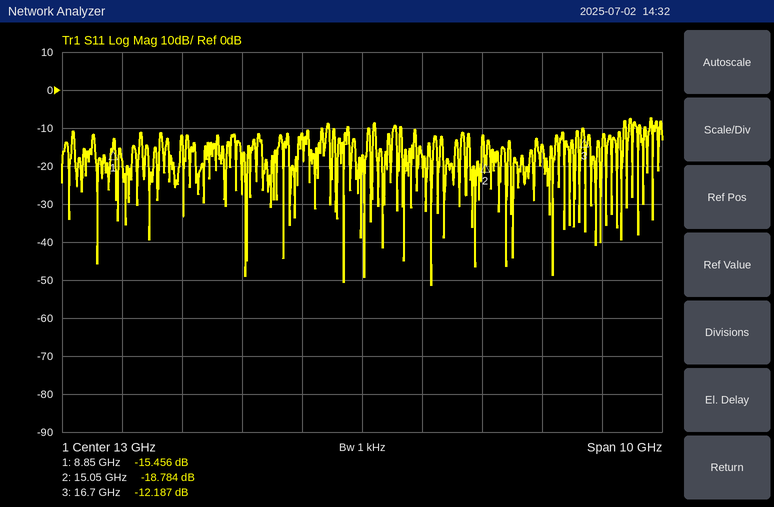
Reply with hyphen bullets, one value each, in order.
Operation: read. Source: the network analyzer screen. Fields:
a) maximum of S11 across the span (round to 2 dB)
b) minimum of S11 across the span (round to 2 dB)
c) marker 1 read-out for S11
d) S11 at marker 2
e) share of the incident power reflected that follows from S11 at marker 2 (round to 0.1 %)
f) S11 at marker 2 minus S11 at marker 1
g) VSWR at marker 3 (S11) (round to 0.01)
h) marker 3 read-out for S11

- -8 dB
- -52 dB
- -15.456 dB
- -18.784 dB
- 1.3 %
- -3.328 dB
- 1.65
- -12.187 dB
